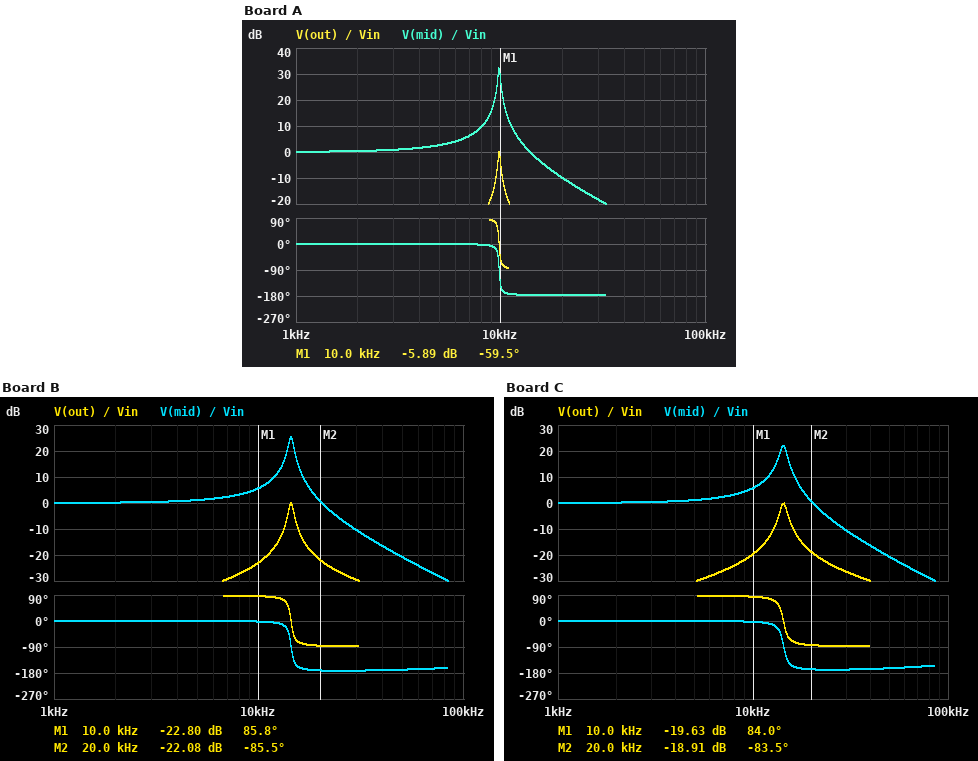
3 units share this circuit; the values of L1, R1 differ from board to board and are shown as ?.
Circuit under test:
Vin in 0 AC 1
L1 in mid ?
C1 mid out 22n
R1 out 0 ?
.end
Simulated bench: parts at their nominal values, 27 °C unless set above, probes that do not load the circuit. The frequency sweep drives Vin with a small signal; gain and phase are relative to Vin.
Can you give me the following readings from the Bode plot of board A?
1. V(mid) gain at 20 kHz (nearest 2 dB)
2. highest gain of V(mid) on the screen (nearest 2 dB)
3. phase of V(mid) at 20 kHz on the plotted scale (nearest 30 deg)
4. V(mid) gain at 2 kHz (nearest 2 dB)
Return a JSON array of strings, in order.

["-10 dB", "32 dB", "-180 deg", "0 dB"]
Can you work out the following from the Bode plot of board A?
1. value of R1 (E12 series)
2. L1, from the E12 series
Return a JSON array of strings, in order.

["18 Ω", "12 mH"]
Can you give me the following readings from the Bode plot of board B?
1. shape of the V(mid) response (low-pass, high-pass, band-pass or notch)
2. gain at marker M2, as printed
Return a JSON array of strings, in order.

["low-pass", "-22.08 dB"]
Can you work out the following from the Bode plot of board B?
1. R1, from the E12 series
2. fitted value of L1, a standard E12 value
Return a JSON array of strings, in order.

["27 Ω", "5.6 mH"]
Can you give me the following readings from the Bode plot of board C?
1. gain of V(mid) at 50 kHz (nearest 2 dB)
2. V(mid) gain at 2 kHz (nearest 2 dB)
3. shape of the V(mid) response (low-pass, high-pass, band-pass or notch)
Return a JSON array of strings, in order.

["-20 dB", "0 dB", "low-pass"]
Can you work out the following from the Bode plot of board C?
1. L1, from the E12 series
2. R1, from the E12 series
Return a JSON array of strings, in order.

["5.6 mH", "39 Ω"]
